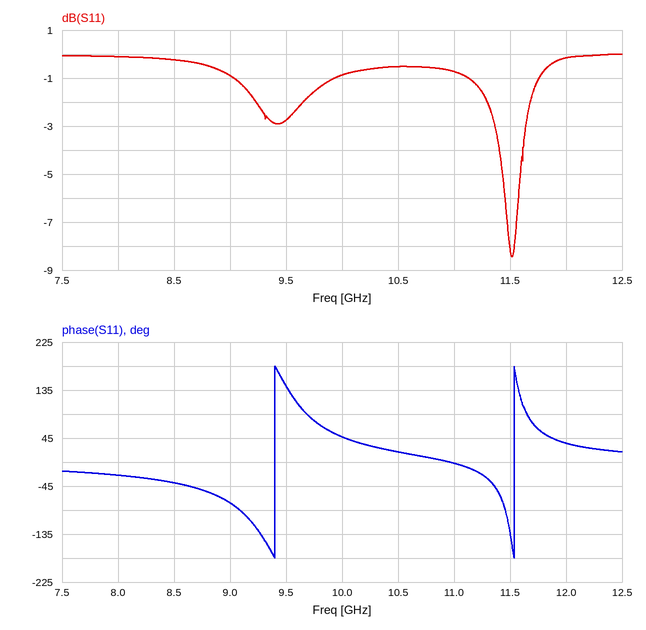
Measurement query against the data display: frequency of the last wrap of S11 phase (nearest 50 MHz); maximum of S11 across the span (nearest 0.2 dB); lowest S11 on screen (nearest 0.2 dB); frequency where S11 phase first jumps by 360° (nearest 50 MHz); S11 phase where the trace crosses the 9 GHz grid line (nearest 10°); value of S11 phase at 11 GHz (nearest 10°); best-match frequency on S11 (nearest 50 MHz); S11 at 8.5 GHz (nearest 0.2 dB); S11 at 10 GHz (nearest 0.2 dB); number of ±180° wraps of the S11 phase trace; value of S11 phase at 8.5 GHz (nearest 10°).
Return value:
11.55 GHz
0.0 dB
-8.4 dB
9.40 GHz
-80°
0°
11.50 GHz
-0.2 dB
-0.8 dB
2
-40°
